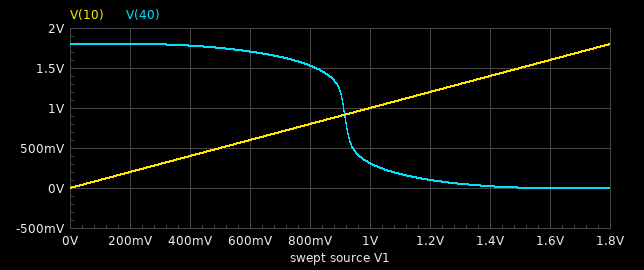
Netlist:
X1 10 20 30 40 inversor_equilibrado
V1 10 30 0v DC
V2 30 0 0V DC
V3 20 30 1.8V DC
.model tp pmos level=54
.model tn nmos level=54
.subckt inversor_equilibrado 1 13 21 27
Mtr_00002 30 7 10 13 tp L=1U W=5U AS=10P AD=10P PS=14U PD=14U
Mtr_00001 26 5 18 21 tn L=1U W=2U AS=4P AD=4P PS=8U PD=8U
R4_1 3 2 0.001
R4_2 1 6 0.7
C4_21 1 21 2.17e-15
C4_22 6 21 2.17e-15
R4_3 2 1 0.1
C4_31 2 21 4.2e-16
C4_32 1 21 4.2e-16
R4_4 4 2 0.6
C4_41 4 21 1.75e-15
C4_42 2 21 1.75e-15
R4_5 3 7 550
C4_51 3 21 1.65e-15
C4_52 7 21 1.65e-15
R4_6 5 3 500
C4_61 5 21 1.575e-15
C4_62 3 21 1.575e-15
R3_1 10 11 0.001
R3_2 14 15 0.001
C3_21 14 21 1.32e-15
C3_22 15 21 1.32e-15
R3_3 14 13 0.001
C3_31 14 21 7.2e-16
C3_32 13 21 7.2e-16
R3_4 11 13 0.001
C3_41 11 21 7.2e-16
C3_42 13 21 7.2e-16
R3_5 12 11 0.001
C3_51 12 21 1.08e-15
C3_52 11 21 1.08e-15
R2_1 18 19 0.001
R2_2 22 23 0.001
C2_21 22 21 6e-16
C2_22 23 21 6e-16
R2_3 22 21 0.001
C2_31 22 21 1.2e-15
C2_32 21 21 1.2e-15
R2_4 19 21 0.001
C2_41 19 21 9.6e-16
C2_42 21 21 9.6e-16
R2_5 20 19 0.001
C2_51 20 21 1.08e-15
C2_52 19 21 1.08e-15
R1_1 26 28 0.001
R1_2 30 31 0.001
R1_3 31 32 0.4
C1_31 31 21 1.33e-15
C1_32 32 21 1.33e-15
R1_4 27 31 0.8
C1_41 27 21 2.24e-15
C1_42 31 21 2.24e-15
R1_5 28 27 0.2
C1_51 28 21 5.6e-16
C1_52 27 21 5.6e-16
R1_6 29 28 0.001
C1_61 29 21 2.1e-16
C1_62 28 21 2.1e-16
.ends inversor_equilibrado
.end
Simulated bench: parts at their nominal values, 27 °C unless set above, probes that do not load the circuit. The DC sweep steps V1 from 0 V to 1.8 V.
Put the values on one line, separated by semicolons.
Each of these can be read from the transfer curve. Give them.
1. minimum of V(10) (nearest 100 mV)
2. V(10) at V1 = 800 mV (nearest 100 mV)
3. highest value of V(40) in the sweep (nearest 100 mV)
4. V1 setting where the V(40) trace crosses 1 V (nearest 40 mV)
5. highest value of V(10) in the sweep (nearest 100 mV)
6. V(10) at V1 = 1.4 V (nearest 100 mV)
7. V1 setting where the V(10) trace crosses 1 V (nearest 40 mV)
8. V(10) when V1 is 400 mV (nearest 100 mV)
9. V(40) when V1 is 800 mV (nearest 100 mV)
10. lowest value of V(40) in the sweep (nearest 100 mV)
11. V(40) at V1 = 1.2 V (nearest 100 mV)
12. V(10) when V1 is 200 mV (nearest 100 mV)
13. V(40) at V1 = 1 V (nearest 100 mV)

0 V; 800 mV; 1.8 V; 920 mV; 1.8 V; 1.4 V; 1.00 V; 400 mV; 1.5 V; 0 V; 100 mV; 200 mV; 300 mV
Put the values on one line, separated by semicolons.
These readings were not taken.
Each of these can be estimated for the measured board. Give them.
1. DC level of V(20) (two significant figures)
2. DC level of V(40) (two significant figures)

1.8 V; 1.8 V
